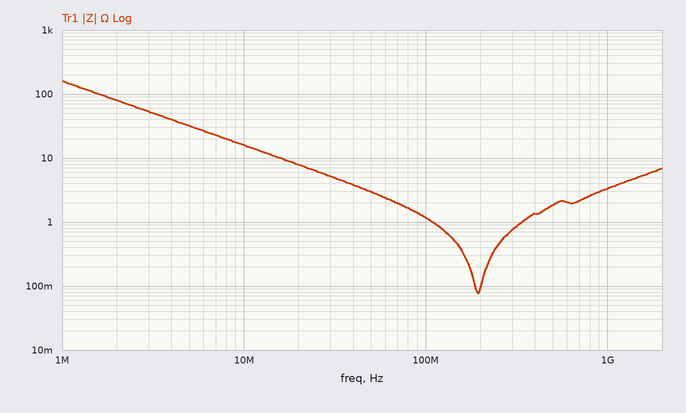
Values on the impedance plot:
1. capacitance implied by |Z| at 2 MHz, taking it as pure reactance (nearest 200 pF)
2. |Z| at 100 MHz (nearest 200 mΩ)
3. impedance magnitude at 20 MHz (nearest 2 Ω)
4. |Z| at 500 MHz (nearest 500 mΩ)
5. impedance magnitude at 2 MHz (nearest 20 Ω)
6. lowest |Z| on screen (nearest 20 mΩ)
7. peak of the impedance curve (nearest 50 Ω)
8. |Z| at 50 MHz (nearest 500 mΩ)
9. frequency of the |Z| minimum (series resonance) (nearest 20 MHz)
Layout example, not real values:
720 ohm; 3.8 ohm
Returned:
1.0 nF; 1.2 Ω; 8 Ω; 2.0 Ω; 80 Ω; 80 mΩ; 150 Ω; 3.0 Ω; 200 MHz
